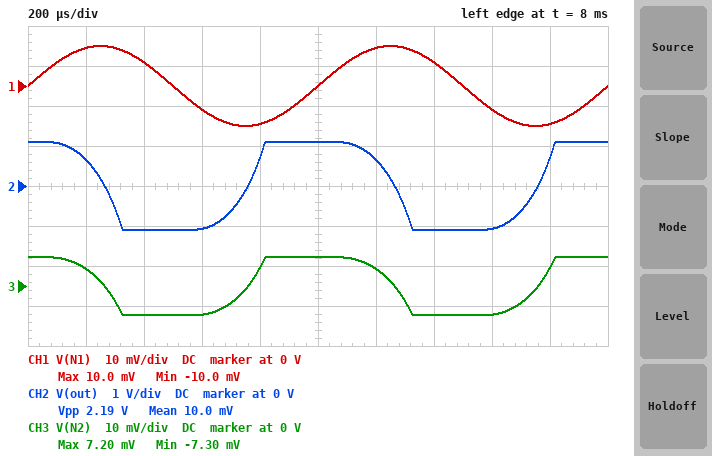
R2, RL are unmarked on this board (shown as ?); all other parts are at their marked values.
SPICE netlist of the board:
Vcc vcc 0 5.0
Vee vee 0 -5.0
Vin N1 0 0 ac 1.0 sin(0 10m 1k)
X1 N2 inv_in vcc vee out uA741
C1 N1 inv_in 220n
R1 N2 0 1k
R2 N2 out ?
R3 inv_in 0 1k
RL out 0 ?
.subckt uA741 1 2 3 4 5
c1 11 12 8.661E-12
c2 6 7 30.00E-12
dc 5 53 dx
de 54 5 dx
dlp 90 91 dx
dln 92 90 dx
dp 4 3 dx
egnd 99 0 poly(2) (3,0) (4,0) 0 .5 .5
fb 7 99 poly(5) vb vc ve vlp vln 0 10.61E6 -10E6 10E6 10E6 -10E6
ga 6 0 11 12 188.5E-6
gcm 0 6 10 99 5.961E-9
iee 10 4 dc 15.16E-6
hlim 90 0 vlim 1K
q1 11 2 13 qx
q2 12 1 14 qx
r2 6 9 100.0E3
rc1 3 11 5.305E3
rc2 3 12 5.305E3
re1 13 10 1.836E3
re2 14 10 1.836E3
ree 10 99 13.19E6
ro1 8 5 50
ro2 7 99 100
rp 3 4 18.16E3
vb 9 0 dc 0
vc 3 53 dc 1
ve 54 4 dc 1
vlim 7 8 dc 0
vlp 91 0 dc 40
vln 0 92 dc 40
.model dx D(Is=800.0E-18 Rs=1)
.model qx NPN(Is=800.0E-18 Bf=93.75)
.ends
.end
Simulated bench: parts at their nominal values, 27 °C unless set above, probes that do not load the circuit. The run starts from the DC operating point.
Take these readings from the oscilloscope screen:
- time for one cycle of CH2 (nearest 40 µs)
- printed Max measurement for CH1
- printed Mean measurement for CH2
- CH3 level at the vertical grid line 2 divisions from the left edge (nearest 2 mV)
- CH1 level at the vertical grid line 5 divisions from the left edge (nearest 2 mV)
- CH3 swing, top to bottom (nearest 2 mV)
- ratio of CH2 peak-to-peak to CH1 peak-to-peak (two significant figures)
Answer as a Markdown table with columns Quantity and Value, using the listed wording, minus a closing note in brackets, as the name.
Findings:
| Quantity | Value |
|---|---|
| time for one cycle of CH2 | 1.00 ms |
| printed Max measurement for CH1 | 10.0 mV |
| printed Mean measurement for CH2 | 10.0 mV |
| CH3 level at the vertical grid line 2 divisions from the left edge | -8 mV |
| CH1 level at the vertical grid line 5 divisions from the left edge | 0 V |
| CH3 swing, top to bottom | 14 mV |
| ratio of CH2 peak-to-peak to CH1 peak-to-peak | 110 |
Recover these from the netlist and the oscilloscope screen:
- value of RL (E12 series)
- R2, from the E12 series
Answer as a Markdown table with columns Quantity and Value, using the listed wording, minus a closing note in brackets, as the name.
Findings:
| Quantity | Value |
|---|---|
| value of RL | 27 Ω |
| R2, from the E12 series | 150 kΩ |
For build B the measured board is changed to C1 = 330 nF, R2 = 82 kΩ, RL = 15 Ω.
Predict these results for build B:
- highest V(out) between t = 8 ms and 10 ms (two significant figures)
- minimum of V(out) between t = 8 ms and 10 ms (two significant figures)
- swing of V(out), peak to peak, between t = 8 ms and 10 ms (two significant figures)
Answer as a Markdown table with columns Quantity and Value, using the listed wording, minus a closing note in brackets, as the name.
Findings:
| Quantity | Value |
|---|---|
| highest V(out) between t = 8 ms and 10 ms | 610 mV |
| minimum of V(out) between t = 8 ms and 10 ms | -610 mV |
| swing of V(out), peak to peak, between t = 8 ms and 10 ms | 1.2 V |
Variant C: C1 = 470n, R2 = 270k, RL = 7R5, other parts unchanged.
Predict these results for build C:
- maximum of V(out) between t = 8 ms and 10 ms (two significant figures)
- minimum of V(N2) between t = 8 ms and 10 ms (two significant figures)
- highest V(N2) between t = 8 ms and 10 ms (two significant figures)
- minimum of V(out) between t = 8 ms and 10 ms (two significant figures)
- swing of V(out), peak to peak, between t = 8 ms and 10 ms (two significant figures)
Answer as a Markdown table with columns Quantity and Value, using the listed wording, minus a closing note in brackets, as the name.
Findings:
| Quantity | Value |
|---|---|
| maximum of V(out) between t = 8 ms and 10 ms | 300 mV |
| minimum of V(N2) between t = 8 ms and 10 ms | -1.2 mV |
| highest V(N2) between t = 8 ms and 10 ms | 1.0 mV |
| minimum of V(out) between t = 8 ms and 10 ms | -300 mV |
| swing of V(out), peak to peak, between t = 8 ms and 10 ms | 610 mV |
